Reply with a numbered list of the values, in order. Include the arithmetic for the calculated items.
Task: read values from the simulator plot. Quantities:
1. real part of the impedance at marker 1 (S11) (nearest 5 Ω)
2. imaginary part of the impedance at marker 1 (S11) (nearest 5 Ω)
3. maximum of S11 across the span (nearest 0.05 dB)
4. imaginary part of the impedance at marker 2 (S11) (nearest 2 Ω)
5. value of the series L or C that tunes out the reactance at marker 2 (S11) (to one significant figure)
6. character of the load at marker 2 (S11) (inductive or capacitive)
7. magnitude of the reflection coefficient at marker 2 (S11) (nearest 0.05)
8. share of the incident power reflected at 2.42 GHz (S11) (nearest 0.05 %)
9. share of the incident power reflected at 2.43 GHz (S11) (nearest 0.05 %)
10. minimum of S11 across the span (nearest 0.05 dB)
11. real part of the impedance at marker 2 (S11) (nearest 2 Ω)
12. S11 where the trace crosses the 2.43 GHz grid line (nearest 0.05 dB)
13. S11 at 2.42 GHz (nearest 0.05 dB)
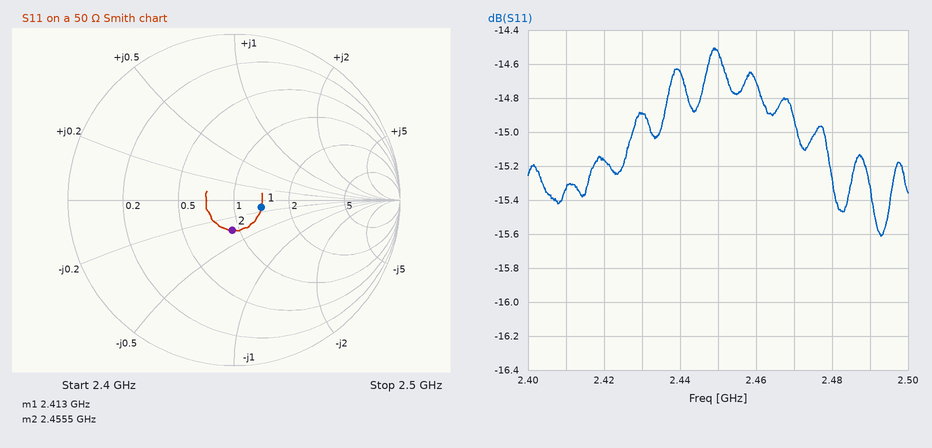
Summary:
1. 70 Ω
2. -5 Ω
3. -14.50 dB
4. -18 Ω
5. L = 18 Ω/(2π × 2.4555 GHz) ≈ 1 nH
6. capacitive
7. 0.20
8. 10^(-15.15/10) ≈ 3.05 %
9. 10^(-14.9/10) ≈ 3.24 %, so 3.25 % to the nearest 0.05 %
10. -15.60 dB
11. 46 Ω
12. -14.90 dB
13. -15.15 dB
